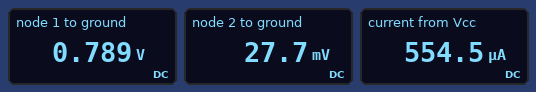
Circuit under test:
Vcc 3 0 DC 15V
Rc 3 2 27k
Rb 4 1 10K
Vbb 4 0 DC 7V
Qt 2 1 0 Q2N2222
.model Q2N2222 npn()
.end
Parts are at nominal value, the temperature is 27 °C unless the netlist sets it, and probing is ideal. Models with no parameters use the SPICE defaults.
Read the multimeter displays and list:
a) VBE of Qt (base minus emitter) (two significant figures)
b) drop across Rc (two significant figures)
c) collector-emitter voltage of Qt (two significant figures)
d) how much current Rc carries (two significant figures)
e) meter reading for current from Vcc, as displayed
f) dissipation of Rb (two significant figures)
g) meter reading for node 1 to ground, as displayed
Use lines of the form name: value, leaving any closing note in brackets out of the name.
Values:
VBE of Qt (base minus emitter): 790 mV
drop across Rc: 15 V
collector-emitter voltage of Qt: 28 mV
how much current Rc carries: 550 µA
meter reading for current from Vcc, as displayed: 554.5 µA
dissipation of Rb: 3.9 mW
meter reading for node 1 to ground, as displayed: 0.789 V
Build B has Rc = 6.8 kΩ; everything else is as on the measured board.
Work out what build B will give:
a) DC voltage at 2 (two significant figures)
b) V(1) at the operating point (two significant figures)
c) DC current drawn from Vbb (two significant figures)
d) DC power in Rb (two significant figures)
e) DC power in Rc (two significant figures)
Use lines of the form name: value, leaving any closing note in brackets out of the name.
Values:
DC voltage at 2: 45 mV
V(1) at the operating point: 810 mV
DC current drawn from Vbb: 620 µA
DC power in Rb: 3.8 mW
DC power in Rc: 33 mW
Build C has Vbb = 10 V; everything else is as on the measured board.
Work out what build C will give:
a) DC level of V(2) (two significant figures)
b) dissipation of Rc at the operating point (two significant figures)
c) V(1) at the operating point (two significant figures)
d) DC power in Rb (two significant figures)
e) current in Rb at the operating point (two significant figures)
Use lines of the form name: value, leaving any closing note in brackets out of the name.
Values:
DC level of V(2): 25 mV
dissipation of Rc at the operating point: 8.3 mW
V(1) at the operating point: 800 mV
DC power in Rb: 8.5 mW
current in Rb at the operating point: 920 µA
